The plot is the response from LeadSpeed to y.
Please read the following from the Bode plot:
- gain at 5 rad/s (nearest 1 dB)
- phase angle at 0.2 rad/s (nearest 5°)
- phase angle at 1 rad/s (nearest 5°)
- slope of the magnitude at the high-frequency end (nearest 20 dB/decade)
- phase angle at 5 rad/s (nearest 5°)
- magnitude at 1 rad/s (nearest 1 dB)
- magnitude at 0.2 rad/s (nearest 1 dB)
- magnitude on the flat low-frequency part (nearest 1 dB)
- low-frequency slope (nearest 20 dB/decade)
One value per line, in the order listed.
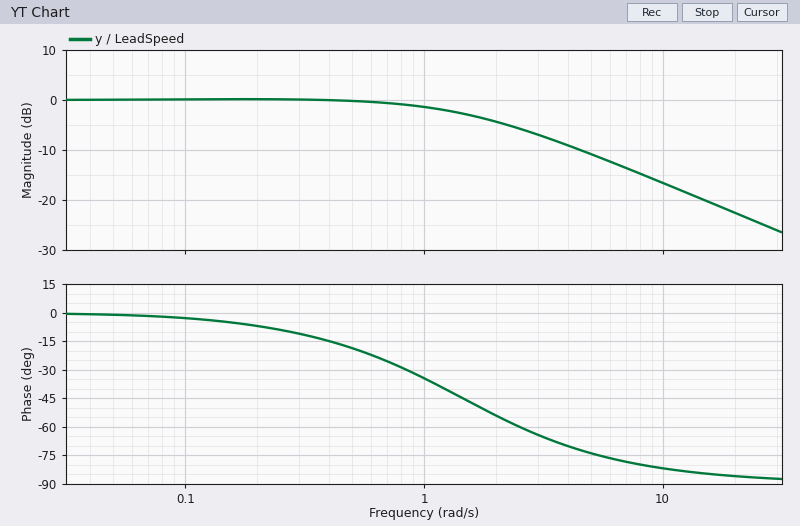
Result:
-11 dB
-5°
-35°
-20 dB/decade
-75°
-1 dB
0 dB
0 dB
0 dB/decade
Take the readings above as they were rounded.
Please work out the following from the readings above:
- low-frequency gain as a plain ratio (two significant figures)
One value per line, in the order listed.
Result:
1.0
